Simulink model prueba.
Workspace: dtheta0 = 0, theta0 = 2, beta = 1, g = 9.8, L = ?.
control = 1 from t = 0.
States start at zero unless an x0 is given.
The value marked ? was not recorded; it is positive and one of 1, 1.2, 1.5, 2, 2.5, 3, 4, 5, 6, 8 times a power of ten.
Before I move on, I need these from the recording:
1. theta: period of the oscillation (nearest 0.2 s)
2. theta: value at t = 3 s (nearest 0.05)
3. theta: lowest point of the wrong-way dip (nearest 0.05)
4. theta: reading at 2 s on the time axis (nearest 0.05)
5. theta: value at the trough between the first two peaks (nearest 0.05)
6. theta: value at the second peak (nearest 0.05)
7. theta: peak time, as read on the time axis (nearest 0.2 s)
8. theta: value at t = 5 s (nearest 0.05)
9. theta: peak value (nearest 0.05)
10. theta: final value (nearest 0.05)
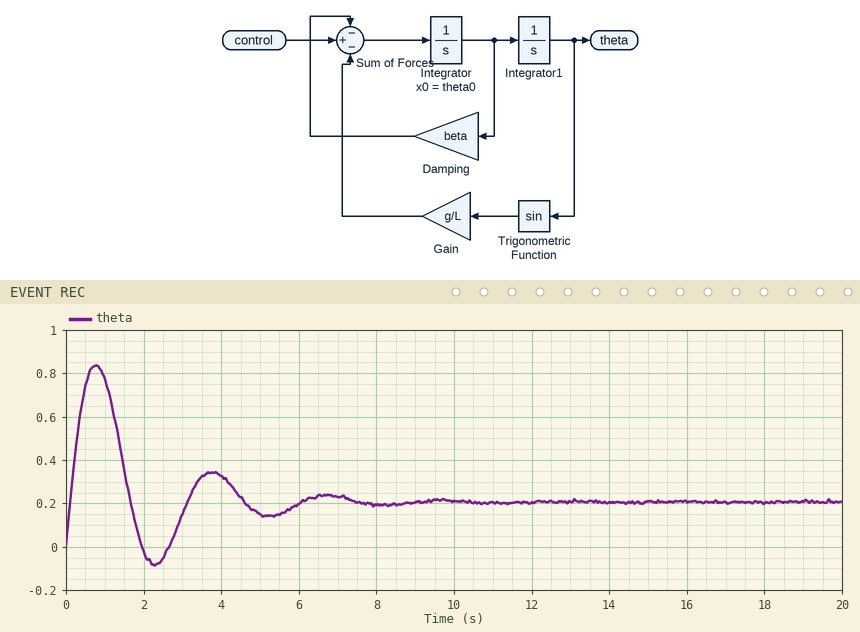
3.0 s
0.15
-0.10
0.00
-0.10
0.35
0.8 s
0.15
0.85
0.20
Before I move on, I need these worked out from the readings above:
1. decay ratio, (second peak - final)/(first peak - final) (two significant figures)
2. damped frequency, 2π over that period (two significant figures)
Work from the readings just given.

0.23
2.1 rad/s
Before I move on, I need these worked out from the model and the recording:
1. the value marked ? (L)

2
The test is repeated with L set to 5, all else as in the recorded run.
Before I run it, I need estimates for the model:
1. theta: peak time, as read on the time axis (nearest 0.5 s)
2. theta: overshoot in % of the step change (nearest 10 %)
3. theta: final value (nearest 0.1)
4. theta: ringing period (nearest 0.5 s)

1.5 s
150 %
0.5
5.5 s
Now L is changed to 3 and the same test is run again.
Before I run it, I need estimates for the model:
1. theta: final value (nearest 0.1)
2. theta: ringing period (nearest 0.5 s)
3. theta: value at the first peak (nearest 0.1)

0.3
4.0 s
1.0
